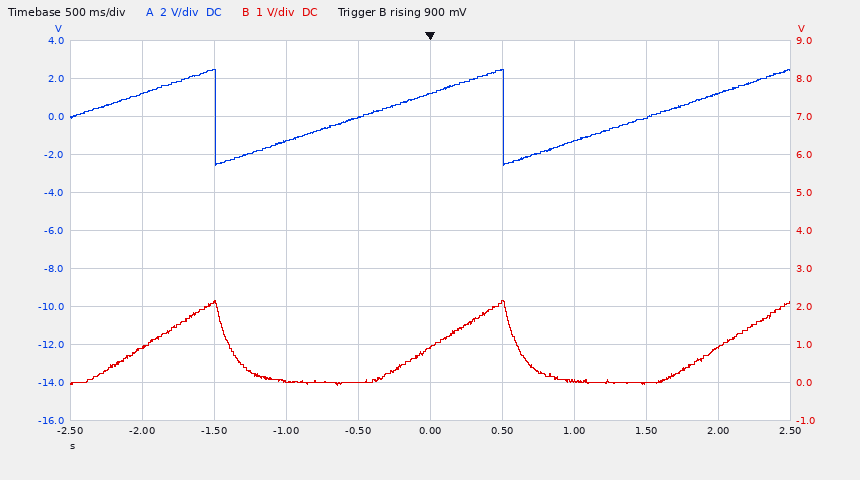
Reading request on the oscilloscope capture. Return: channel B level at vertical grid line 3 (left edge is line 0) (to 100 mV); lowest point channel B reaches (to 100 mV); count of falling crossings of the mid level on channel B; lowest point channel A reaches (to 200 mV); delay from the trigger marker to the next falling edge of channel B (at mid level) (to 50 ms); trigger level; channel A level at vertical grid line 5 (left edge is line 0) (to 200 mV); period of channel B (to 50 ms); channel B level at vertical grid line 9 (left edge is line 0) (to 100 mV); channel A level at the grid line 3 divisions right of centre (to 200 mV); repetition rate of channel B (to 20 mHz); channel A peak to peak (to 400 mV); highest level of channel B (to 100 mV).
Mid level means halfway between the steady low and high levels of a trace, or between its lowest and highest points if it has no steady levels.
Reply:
0.0 V
-100 mV
2
-2.6 V
600 ms
900 mV
1.2 V
2.00 s
900 mV
0.0 V
500 mHz
5.2 V
2.2 V
